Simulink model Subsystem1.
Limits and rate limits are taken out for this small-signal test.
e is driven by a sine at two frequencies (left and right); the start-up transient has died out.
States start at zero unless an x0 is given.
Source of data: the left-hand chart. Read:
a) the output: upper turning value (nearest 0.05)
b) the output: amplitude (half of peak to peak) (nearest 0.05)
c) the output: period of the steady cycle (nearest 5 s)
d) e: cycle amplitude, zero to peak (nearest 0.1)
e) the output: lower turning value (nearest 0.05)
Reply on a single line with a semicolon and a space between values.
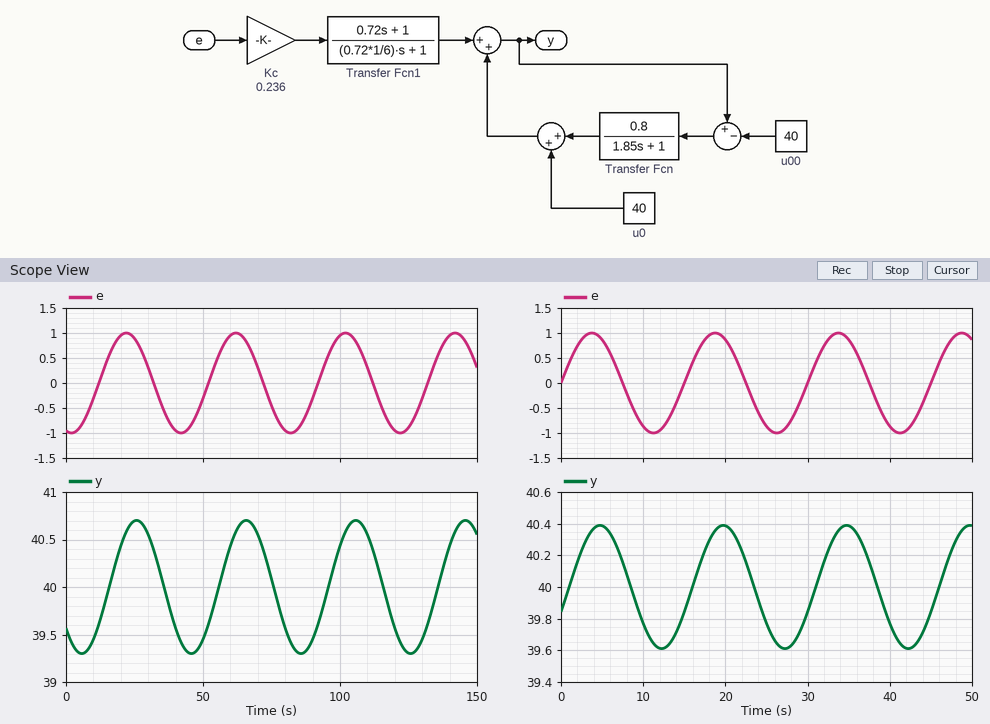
40.70; 0.70; 40 s; 1.0; 39.30
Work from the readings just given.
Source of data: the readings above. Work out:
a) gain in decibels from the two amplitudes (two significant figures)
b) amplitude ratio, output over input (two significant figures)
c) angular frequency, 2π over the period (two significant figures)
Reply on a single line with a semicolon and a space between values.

-3.1 dB; 0.70; 0.16 rad/s
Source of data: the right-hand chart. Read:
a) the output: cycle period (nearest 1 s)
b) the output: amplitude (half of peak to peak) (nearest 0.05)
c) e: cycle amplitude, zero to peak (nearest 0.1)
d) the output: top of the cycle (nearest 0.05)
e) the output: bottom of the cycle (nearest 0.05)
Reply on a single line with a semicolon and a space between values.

15 s; 0.40; 1.0; 40.40; 39.60
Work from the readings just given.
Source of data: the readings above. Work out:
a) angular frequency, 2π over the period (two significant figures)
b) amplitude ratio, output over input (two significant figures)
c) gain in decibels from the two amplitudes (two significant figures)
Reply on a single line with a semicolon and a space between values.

0.42 rad/s; 0.40; -8.0 dB
